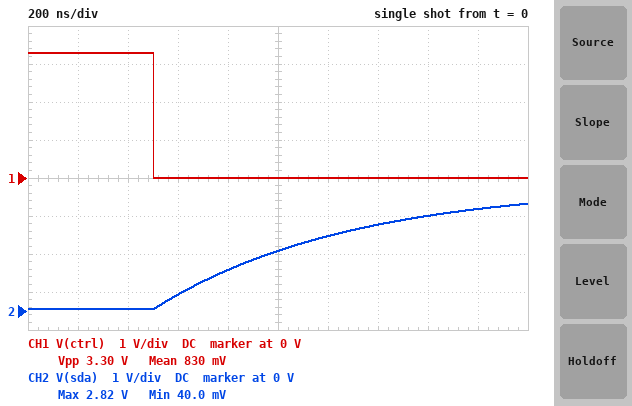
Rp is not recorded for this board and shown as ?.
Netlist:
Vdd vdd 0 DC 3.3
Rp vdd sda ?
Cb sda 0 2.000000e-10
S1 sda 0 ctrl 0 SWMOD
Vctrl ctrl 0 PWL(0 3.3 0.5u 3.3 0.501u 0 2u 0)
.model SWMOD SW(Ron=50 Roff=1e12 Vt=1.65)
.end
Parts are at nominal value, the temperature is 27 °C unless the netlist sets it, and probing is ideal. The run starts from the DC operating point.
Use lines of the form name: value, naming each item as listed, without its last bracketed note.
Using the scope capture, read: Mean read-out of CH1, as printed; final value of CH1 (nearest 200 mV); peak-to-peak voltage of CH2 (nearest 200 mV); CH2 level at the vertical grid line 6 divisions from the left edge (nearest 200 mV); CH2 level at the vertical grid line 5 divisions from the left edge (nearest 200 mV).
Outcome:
Mean read-out of CH1, as printed: 830 mV
final value of CH1: 0 V
peak-to-peak voltage of CH2: 2.8 V
CH2 level at the vertical grid line 6 divisions from the left edge: 2.0 V
CH2 level at the vertical grid line 5 divisions from the left edge: 1.6 V
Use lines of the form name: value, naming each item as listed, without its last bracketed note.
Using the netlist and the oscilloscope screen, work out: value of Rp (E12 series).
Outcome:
value of Rp: 3.9 kΩ
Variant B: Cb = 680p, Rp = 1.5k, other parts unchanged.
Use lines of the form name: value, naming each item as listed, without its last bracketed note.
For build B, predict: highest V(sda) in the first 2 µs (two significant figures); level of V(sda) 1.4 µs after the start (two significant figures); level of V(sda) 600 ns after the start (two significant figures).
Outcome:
highest V(sda) in the first 2 µs: 2.6 V
level of V(sda) 1.4 µs after the start: 2.0 V
level of V(sda) 600 ns after the start: 400 mV
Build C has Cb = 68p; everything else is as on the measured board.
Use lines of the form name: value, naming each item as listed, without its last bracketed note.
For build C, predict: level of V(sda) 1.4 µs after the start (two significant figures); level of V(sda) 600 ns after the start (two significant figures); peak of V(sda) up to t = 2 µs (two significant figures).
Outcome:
level of V(sda) 1.4 µs after the start: 3.2 V
level of V(sda) 600 ns after the start: 1.1 V
peak of V(sda) up to t = 2 µs: 3.3 V
